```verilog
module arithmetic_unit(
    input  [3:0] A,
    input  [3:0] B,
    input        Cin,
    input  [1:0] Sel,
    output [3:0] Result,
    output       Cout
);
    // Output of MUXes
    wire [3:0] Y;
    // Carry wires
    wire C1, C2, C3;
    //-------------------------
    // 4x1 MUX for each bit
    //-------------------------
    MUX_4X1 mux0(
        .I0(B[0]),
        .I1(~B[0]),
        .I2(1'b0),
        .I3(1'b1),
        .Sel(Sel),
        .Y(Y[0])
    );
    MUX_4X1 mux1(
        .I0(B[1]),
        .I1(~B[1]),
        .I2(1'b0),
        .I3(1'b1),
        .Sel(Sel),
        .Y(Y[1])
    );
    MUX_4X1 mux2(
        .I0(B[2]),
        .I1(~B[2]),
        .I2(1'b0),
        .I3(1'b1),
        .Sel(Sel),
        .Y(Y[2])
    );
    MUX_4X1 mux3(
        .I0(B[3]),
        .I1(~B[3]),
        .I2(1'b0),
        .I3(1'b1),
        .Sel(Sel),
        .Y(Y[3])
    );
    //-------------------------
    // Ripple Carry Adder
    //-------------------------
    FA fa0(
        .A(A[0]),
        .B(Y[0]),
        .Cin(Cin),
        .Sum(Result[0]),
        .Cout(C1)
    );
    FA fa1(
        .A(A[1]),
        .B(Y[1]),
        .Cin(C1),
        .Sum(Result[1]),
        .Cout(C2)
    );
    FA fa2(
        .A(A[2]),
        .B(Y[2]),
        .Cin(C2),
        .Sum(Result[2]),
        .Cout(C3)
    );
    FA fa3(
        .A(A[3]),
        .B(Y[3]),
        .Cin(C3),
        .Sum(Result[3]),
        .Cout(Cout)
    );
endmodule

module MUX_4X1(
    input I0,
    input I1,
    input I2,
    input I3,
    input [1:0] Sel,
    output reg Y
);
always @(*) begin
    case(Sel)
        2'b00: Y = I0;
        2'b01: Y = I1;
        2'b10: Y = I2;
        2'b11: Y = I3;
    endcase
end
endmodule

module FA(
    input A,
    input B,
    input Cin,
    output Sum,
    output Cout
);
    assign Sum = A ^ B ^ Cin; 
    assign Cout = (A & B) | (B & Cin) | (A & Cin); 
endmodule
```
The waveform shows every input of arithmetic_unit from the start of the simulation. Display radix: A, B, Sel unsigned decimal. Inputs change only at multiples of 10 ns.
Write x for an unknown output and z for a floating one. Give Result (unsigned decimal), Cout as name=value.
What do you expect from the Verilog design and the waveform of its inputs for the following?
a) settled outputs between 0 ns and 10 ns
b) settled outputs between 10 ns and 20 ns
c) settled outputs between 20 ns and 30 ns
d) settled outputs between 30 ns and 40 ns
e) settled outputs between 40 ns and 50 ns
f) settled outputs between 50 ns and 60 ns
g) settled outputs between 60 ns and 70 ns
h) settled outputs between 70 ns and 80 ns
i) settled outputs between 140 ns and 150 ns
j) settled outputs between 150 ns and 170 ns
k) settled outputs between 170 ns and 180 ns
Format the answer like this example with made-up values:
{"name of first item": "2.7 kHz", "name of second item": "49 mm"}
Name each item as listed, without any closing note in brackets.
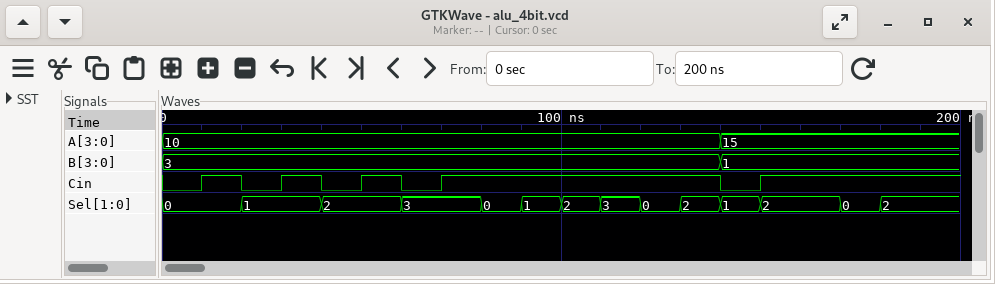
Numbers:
{"settled outputs between 0 ns and 10 ns": "Result=13, Cout=0", "settled outputs between 10 ns and 20 ns": "Result=14, Cout=0", "settled outputs between 20 ns and 30 ns": "Result=6, Cout=1", "settled outputs between 30 ns and 40 ns": "Result=7, Cout=1", "settled outputs between 40 ns and 50 ns": "Result=10, Cout=0", "settled outputs between 50 ns and 60 ns": "Result=11, Cout=0", "settled outputs between 60 ns and 70 ns": "Result=9, Cout=1", "settled outputs between 70 ns and 80 ns": "Result=10, Cout=1", "settled outputs between 140 ns and 150 ns": "Result=13, Cout=1", "settled outputs between 150 ns and 170 ns": "Result=0, Cout=1", "settled outputs between 170 ns and 180 ns": "Result=1, Cout=1"}
